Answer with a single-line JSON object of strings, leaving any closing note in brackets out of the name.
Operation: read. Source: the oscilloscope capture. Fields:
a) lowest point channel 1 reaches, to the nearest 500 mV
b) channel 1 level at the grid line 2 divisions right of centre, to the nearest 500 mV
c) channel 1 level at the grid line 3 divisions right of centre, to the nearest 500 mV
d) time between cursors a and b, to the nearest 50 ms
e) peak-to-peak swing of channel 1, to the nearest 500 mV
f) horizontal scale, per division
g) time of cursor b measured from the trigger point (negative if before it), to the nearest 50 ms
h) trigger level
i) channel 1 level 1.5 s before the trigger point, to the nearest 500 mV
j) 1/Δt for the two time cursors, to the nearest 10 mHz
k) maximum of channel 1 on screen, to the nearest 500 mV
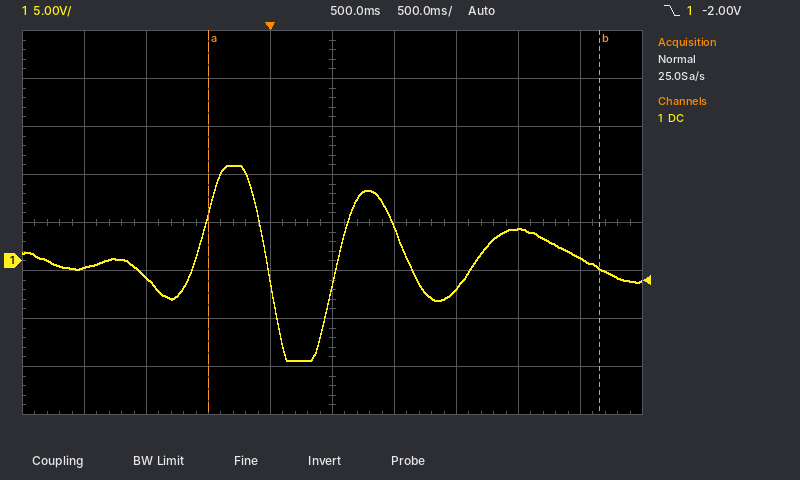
{"lowest point channel 1 reaches, to the nearest 500 mV": "-10.5 V", "channel 1 level at the grid line 2 divisions right of centre, to the nearest 500 mV": "-3.0 V", "channel 1 level at the grid line 3 divisions right of centre, to the nearest 500 mV": "3.5 V", "time between cursors a and b, to the nearest 50 ms": "3.15 s", "peak-to-peak swing of channel 1, to the nearest 500 mV": "20.5 V", "horizontal scale, per division": "500 ms", "time of cursor b measured from the trigger point (negative if before it), to the nearest 50 ms": "+2.65 s", "trigger level": "-2.00 V", "channel 1 level 1.5 s before the trigger point, to the nearest 500 mV": "-500 mV", "1/Δt for the two time cursors, to the nearest 10 mHz": "320 mHz", "maximum of channel 1 on screen, to the nearest 500 mV": "10.0 V"}
